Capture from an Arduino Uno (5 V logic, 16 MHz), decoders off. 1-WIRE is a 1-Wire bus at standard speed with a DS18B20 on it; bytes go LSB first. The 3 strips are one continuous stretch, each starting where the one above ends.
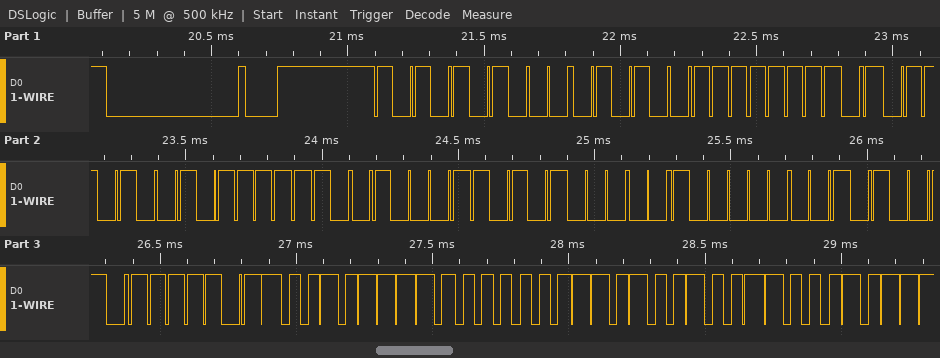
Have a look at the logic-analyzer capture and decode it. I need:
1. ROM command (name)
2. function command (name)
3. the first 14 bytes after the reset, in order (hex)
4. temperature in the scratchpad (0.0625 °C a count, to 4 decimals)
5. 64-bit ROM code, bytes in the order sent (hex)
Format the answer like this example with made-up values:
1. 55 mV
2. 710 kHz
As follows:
1. Match ROM
2. Read Scratchpad
3. 55 28 FF 5A FA 89 15 04 94 BE E9 01 4B 46
4. 30.5625 °C
5. 28 FF 5A FA 89 15 04 94
